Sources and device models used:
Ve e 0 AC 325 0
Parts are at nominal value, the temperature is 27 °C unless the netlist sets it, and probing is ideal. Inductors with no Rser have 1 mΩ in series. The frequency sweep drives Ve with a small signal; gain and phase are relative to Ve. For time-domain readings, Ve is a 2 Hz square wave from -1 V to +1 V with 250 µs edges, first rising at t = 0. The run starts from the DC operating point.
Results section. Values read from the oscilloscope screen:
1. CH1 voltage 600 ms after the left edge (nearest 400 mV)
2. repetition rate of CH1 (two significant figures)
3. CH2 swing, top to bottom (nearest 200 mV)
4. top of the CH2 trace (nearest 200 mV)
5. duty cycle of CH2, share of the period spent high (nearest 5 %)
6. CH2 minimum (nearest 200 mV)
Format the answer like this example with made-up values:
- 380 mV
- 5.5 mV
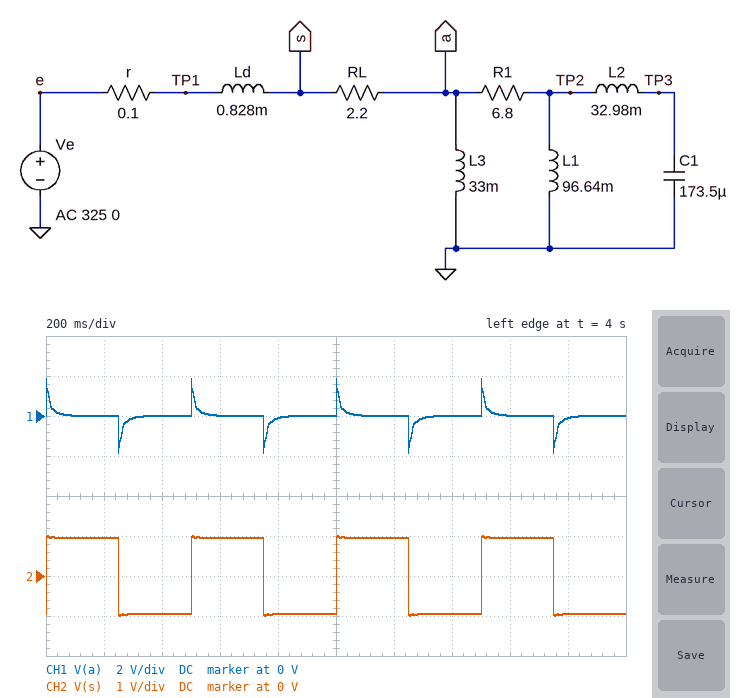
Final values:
- 0 V
- 2.0 Hz
- 2.0 V
- 1.0 V
- 50 %
- -1.0 V
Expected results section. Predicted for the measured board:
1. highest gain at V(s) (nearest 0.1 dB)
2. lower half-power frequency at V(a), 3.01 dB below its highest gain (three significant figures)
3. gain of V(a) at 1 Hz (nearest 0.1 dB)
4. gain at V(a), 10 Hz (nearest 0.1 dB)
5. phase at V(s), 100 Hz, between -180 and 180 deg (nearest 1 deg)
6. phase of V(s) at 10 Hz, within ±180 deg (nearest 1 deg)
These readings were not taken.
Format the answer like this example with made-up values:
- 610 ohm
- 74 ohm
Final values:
- -0.1 dB
- 13.9 Hz
- -21.0 dB
- -4.9 dB
- -1 deg
- 0 deg
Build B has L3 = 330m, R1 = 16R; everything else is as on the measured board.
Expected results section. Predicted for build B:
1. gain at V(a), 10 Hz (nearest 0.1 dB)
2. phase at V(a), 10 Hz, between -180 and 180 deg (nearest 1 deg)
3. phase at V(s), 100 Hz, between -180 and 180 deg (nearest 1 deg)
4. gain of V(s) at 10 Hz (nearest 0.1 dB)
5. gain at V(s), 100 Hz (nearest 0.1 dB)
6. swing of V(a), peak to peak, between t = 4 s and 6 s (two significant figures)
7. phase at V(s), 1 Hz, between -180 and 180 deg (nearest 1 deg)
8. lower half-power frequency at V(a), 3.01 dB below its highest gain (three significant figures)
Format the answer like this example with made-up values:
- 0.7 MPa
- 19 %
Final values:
- -1.1 dB
- 8 deg
- -1 deg
- -0.1 dB
- -0.2 dB
- 3.2 V
- 1 deg
- 1.34 Hz
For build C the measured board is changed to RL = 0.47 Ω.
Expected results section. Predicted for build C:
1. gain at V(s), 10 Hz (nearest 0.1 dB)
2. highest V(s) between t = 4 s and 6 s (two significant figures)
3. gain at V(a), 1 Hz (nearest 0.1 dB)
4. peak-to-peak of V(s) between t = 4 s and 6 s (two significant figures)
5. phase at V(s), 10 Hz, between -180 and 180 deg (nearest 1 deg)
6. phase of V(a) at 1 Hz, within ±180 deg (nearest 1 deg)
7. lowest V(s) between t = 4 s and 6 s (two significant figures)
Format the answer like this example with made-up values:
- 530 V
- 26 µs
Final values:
- -0.4 dB
- 1.1 V
- -9.5 dB
- 2.2 V
- 2 deg
- 68 deg
- -1.1 V
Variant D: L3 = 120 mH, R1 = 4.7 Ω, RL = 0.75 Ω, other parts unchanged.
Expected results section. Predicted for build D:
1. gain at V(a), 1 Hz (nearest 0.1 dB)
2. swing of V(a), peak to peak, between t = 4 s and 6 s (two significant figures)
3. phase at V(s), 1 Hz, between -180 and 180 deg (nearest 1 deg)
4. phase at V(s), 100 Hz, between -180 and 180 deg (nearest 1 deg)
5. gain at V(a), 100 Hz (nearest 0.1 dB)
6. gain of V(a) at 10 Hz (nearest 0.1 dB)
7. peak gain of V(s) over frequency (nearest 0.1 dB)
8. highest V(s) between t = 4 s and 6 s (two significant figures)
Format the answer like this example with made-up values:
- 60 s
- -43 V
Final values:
- -4.4 dB
- 3.2 V
- 3 deg
- -1 deg
- -0.7 dB
- -0.8 dB
- 0.1 dB
- 1.1 V
